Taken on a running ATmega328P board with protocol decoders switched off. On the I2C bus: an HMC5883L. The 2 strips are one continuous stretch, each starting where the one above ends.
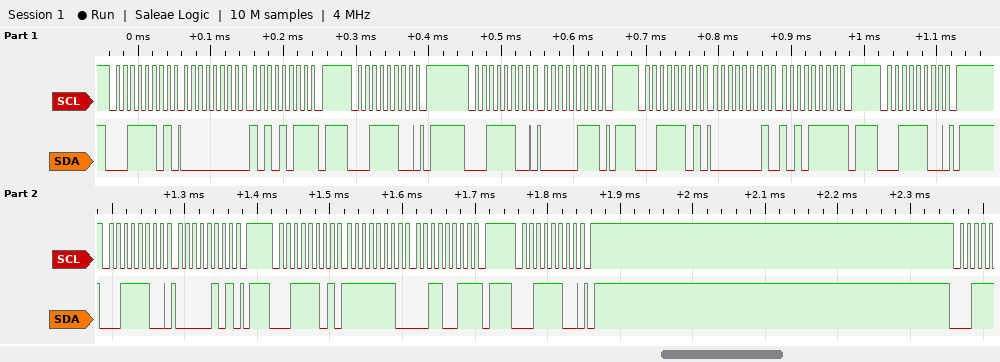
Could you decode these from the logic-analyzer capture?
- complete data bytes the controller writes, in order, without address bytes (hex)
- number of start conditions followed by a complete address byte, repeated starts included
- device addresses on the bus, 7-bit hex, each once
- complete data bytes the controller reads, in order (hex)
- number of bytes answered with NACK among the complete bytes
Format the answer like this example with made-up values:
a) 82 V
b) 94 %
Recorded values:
a) 07 05
b) 8
c) 0x1E
d) 00 AB 01 AF FE 33
e) 3
